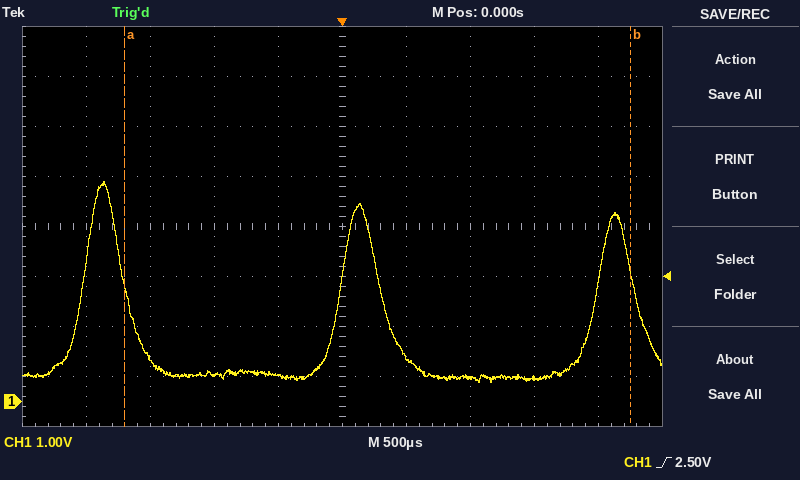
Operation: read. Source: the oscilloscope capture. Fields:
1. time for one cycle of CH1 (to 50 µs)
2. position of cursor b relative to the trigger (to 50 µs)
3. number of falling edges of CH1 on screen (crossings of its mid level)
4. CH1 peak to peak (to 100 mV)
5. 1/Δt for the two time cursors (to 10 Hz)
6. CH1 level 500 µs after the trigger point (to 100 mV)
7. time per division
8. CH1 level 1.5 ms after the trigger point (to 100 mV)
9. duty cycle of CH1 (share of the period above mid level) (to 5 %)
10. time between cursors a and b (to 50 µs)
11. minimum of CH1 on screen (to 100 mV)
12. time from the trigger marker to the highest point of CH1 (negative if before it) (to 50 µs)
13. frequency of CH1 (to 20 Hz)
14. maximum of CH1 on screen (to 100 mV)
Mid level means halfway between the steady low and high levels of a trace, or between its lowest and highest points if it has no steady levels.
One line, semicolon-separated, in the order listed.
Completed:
2.00 ms; +2.25 ms; 3; 4.0 V; 250 Hz; 900 mV; 500 µs; 500 mV; 15 %; 3.95 ms; 400 mV; -1.85 ms; 500 Hz; 4.4 V
